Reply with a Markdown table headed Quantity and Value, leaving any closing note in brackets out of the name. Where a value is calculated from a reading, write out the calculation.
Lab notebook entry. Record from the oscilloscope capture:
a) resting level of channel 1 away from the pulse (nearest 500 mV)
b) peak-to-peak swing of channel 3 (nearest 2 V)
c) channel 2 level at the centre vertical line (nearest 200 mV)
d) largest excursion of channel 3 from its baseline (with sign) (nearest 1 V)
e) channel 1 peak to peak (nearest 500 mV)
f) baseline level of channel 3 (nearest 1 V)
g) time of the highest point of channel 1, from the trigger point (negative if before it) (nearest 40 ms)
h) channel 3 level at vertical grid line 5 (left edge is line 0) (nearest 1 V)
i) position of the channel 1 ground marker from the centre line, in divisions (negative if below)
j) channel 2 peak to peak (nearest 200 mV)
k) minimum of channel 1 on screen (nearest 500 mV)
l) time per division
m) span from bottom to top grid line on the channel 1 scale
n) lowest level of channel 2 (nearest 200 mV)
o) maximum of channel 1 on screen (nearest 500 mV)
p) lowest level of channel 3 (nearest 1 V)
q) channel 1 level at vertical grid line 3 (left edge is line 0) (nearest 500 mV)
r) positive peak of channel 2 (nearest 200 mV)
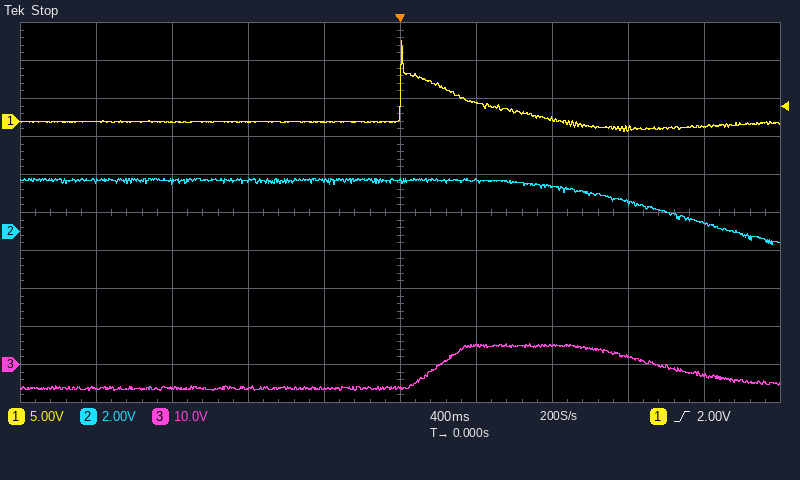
| Quantity | Value |
|---|---|
| resting level of channel 1 away from the pulse | 0.0 V |
| peak-to-peak swing of channel 3 | 12 V |
| channel 2 level at the centre vertical line | 2.6 V |
| largest excursion of channel 3 from its baseline (with sign) | +12 V |
| channel 1 peak to peak | 10.5 V − (-1.5 V) = 12.0 V |
| baseline level of channel 3 | -6 V |
| time of the highest point of channel 1, from the trigger point (negative if before it) | 0 ms |
| channel 3 level at vertical grid line 5 (left edge is line 0) | -6 V |
| position of the channel 1 ground marker from the centre line, in divisions | +2.4 div |
| channel 2 peak to peak | 2.8 V − (-600 mV) = 3.4 V |
| minimum of channel 1 on screen | -1.5 V |
| time per division | 400 ms |
| span from bottom to top grid line on the channel 1 scale | 50 V |
| lowest level of channel 2 | -600 mV |
| maximum of channel 1 on screen | 10.5 V |
| lowest level of channel 3 | -7 V |
| channel 1 level at vertical grid line 3 (left edge is line 0) | 0.0 V |
| positive peak of channel 2 | 2.8 V |
